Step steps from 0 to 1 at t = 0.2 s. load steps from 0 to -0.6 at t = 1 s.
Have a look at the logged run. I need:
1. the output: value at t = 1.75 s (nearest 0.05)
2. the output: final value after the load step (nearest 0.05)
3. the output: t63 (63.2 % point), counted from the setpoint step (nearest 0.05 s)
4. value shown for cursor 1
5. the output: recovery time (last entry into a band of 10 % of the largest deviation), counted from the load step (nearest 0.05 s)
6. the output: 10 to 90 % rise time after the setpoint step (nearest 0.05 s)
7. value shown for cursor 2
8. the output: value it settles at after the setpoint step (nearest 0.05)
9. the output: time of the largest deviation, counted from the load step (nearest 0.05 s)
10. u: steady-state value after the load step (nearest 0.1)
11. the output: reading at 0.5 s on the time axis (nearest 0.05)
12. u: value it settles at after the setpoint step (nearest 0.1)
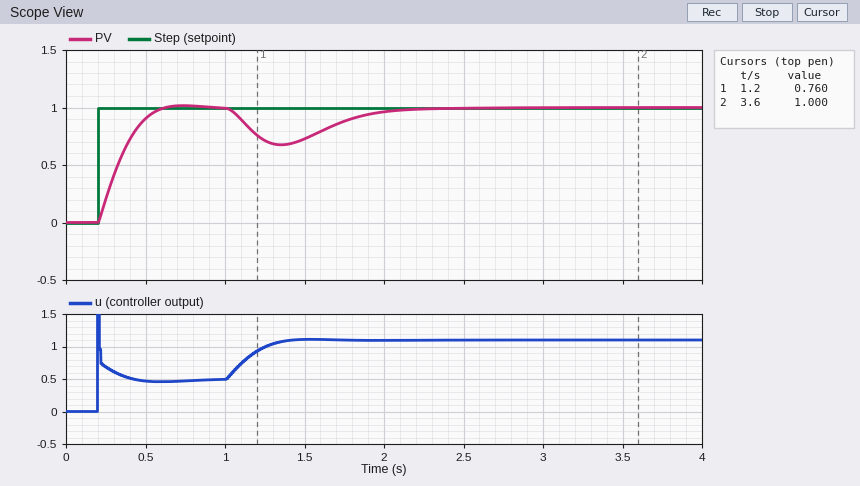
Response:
0.90
1.00
0.15 s
0.760
1.05 s
0.25 s
1.000
1.00
0.35 s
1.1
0.90
0.5
